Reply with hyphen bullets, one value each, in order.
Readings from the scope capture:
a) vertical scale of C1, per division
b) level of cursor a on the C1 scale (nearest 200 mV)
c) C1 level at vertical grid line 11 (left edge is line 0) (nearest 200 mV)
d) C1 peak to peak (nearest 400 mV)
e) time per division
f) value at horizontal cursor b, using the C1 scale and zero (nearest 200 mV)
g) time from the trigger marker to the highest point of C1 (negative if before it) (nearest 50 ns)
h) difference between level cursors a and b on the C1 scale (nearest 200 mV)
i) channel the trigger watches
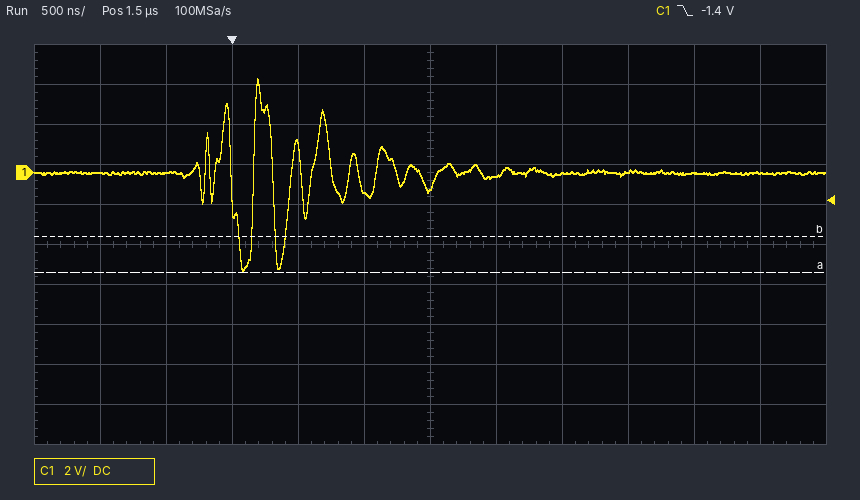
- 2 V
- -5.0 V
- 0.0 V
- 9.6 V
- 500 ns
- -3.2 V
- +200 ns
- 1.8 V
- C1
